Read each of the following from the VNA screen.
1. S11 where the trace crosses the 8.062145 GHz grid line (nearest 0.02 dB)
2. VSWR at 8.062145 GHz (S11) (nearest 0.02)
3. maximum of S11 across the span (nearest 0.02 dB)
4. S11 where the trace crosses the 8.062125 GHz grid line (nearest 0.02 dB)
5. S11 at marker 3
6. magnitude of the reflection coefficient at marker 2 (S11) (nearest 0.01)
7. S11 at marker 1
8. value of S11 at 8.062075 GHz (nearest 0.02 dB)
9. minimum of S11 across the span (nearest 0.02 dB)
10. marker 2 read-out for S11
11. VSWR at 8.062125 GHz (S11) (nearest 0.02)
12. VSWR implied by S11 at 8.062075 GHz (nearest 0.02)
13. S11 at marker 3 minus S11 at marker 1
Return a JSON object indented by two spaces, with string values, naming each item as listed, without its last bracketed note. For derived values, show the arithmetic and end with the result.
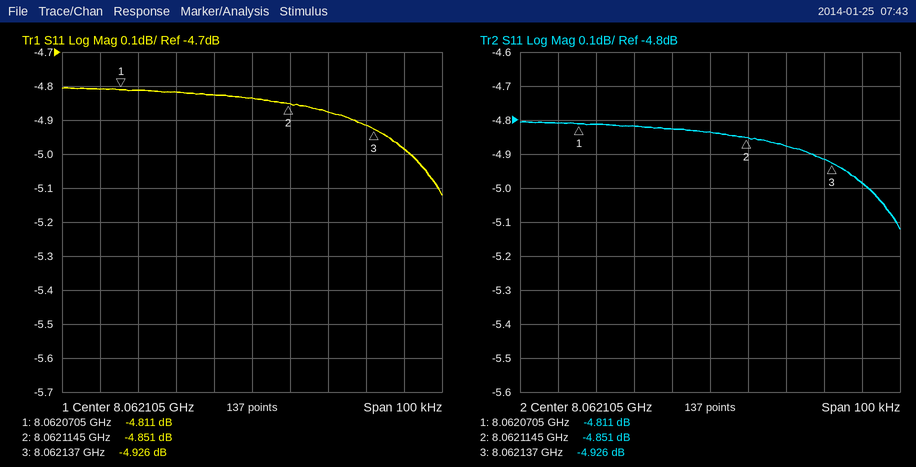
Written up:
{
  "S11 where the trace crosses the 8.062145 GHz grid line": "-4.98 dB",
  "VSWR at 8.062145 GHz (S11)": "|Γ| = 10^(-4.98/20) = 0.5636; VSWR = (1 + 0.5636)/(1 − 0.5636) ≈ 3.58",
  "maximum of S11 across the span": "-4.80 dB",
  "S11 where the trace crosses the 8.062125 GHz grid line": "-4.88 dB",
  "S11 at marker 3": "-4.926 dB",
  "magnitude of the reflection coefficient at marker 2 (S11)": "10^(-4.851/20) ≈ 0.57",
  "S11 at marker 1": "-4.811 dB",
  "value of S11 at 8.062075 GHz": "-4.82 dB",
  "minimum of S11 across the span": "-5.12 dB",
  "marker 2 read-out for S11": "-4.851 dB",
  "VSWR at 8.062125 GHz (S11)": "|Γ| = 10^(-4.88/20) = 0.5702; VSWR = (1 + 0.5702)/(1 − 0.5702) ≈ 3.65, so 3.66 to the nearest 0.02",
  "VSWR implied by S11 at 8.062075 GHz": "|Γ| = 10^(-4.82/20) = 0.5741; VSWR = (1 + 0.5741)/(1 − 0.5741) ≈ 3.70",
  "S11 at marker 3 minus S11 at marker 1": "-4.926 − (-4.811) = -0.115 dB"
}
